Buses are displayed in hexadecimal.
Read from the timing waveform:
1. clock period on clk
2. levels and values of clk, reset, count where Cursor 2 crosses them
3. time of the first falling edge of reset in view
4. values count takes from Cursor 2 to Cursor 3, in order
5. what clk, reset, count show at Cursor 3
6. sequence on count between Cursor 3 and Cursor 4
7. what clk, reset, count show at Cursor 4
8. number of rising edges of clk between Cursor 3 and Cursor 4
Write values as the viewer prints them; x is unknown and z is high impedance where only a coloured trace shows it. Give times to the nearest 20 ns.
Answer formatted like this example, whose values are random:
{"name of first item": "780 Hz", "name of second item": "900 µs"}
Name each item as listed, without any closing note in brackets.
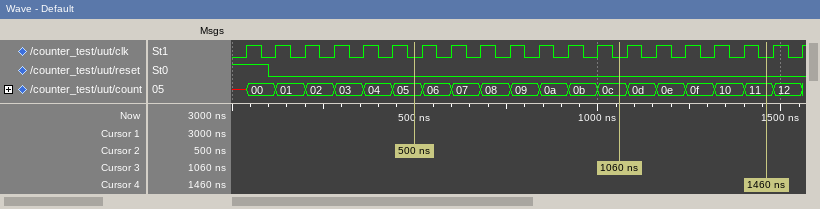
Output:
{"clock period on clk": "80 ns", "levels and values of clk, reset, count where Cursor 2 crosses them": "clk=0, reset=0, count=05", "time of the first falling edge of reset in view": "100 ns", "values count takes from Cursor 2 to Cursor 3, in order": "05, 06, 07, 08, 09, 0a, 0b, 0c", "what clk, reset, count show at Cursor 3": "clk=0, reset=0, count=0c", "sequence on count between Cursor 3 and Cursor 4": "0c, 0d, 0e, 0f, 10, 11", "what clk, reset, count show at Cursor 4": "clk=0, reset=0, count=11", "number of rising edges of clk between Cursor 3 and Cursor 4": "5"}
